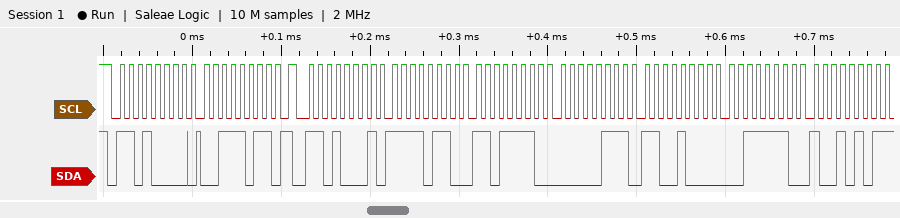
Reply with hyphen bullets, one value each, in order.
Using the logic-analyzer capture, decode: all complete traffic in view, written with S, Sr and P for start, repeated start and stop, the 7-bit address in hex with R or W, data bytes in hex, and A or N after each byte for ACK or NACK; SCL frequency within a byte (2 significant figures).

- S 68W A 3B A Sr 68R A F6 A DE A 07 A C8 A 3E A 95 N
- 100 kHz
